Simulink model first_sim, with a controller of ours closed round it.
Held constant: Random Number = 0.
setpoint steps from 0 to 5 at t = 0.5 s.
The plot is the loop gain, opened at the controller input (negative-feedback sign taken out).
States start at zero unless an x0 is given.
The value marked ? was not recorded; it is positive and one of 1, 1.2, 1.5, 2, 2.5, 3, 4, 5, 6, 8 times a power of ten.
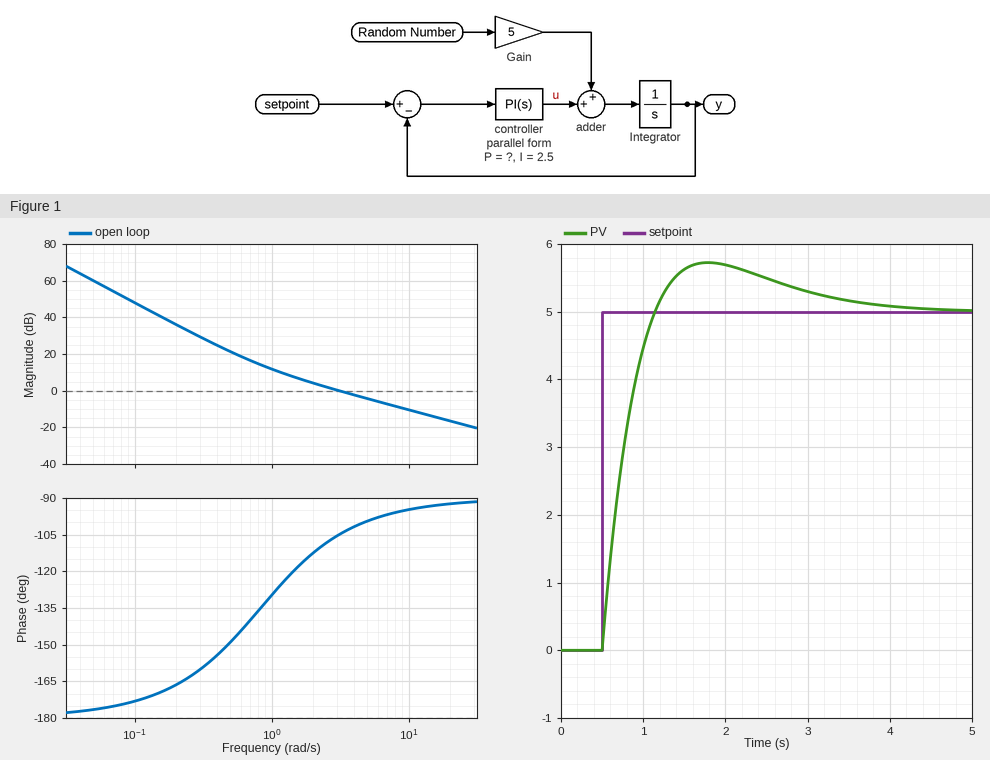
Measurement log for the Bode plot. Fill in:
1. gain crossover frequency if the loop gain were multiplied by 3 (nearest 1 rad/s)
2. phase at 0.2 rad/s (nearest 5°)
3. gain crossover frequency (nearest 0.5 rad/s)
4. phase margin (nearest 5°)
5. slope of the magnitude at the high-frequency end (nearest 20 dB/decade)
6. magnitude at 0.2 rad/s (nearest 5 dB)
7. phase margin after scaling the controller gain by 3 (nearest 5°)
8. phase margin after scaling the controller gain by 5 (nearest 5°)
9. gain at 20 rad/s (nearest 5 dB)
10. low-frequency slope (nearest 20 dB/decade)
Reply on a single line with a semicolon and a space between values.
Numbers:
9 rad/s; -165°; 3.0 rad/s; 75°; -20 dB/decade; 35 dB; 85°; 85°; -15 dB; -40 dB/decade
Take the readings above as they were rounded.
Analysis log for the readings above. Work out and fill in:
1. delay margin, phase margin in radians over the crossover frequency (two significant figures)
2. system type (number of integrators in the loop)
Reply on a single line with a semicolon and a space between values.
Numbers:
0.44 s; 2
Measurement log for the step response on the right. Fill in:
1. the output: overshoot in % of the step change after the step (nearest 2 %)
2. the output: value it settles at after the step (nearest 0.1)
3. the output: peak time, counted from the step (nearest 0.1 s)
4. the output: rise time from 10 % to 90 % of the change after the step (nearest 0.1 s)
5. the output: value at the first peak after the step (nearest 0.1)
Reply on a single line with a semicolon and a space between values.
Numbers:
14 %; 5.0; 1.3 s; 0.5 s; 5.7
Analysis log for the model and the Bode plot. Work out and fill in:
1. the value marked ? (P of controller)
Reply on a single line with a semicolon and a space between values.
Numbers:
3
